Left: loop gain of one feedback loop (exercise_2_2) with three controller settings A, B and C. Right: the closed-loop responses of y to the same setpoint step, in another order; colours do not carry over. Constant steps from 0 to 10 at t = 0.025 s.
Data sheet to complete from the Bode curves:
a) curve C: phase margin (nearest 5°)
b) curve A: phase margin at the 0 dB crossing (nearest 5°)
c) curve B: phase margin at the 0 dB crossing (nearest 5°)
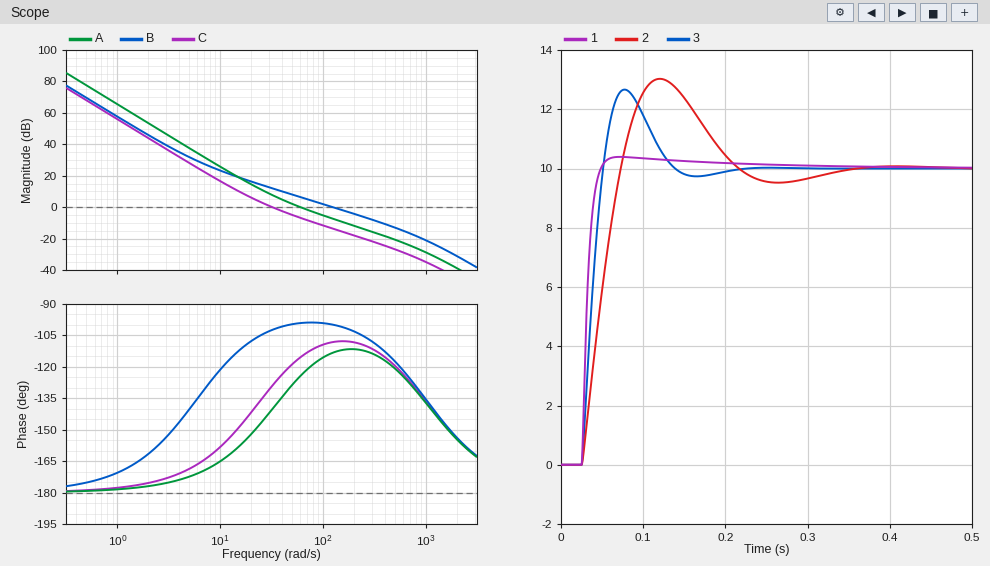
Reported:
50°
55°
80°
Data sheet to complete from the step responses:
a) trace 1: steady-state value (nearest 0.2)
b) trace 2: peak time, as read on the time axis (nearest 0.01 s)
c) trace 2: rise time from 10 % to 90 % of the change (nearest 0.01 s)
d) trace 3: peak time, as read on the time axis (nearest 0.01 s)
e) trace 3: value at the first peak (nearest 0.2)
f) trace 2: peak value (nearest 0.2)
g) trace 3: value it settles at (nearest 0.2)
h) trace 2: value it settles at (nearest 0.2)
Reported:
10.0
0.12 s
0.04 s
0.08 s
12.6
13.0
10.0
10.0
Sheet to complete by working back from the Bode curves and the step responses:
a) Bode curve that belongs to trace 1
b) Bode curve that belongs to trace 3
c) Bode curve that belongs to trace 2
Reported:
B
A
C
